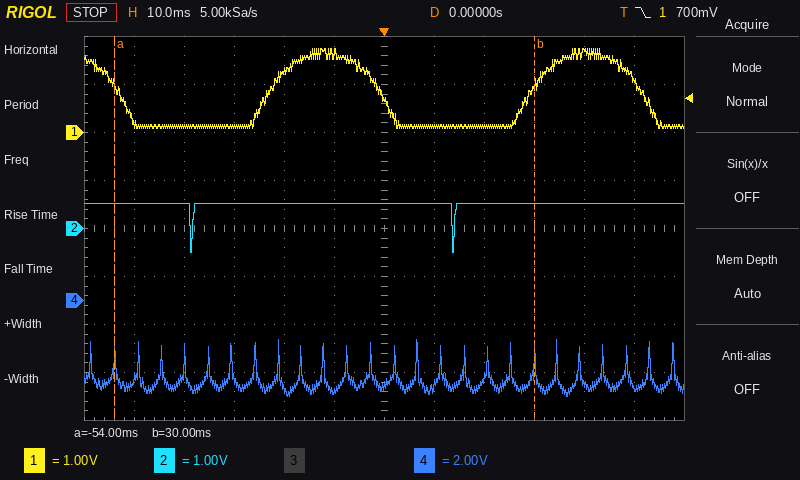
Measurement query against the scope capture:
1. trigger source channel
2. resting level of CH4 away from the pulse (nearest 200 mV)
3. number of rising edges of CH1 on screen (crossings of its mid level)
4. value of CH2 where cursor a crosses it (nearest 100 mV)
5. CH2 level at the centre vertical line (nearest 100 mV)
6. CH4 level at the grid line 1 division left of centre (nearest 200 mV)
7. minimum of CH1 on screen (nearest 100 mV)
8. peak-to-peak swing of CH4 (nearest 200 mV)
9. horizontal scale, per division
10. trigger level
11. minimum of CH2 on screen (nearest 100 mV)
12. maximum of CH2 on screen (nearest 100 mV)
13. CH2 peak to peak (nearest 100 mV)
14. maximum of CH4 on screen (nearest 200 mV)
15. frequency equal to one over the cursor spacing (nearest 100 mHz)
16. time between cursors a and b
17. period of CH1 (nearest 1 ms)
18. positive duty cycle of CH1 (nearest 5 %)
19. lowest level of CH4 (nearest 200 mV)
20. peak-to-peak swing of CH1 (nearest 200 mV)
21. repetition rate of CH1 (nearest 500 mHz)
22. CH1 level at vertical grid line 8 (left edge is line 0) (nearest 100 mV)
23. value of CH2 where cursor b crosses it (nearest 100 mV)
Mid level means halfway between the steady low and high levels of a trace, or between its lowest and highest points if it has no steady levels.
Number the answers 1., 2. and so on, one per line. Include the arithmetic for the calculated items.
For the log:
1. CH1
2. -3.6 V
3. 2
4. 500 mV
5. 500 mV
6. -3.8 V
7. 100 mV
8. -1.6 V − (-4.0 V) = 2.4 V
9. 10 ms
10. 700 mV
11. -500 mV
12. 500 mV
13. 500 mV − (-500 mV) = 1.0 V
14. -1.6 V
15. 1 / 84 ms ≈ 11.9 Hz
16. 30 ms − (-54 ms) = 84 ms
17. 52 ms
18. 40 %
19. -4.0 V
20. 1.6 V
21. 1 / 52 ms ≈ 19.2 Hz, so 19.0 Hz to the nearest 500 mHz
22. 100 mV
23. 500 mV
